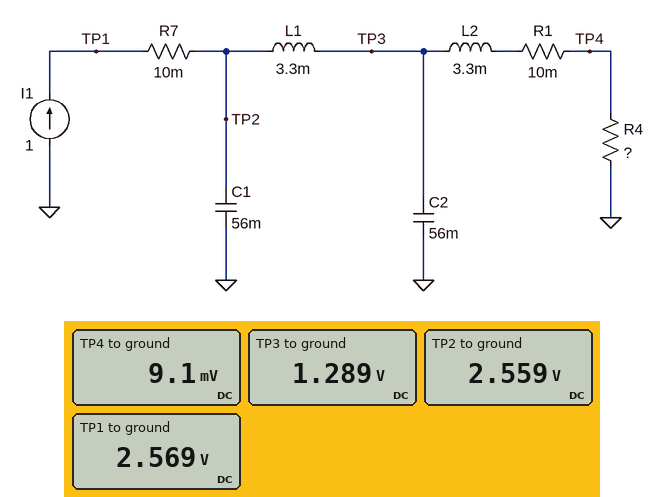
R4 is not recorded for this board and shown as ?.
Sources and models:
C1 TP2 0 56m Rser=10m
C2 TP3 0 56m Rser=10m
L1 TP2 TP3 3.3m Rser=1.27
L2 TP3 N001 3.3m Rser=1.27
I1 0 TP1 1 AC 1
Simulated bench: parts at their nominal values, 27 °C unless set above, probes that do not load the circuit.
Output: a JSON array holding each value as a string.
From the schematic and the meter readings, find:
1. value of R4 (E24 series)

["9.1 mΩ"]
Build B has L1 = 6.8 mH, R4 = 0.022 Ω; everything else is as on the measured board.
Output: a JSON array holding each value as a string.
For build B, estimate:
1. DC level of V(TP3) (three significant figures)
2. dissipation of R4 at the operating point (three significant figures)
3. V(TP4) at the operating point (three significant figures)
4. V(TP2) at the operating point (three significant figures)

["1.30 V", "22.0 mW", "22.0 mV", "2.57 V"]
